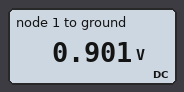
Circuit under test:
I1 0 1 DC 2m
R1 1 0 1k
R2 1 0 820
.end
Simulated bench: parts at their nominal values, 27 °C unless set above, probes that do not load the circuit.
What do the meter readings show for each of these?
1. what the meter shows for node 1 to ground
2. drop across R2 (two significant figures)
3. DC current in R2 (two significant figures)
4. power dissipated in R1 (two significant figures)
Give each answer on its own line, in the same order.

0.901 V
900 mV
1.1 mA
810 µW
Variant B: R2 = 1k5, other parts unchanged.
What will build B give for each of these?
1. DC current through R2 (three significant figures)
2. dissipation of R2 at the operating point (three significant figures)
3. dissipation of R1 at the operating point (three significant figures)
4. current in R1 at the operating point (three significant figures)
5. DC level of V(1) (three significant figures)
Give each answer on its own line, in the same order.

800 µA
960 µW
1.44 mW
1.20 mA
1.20 V
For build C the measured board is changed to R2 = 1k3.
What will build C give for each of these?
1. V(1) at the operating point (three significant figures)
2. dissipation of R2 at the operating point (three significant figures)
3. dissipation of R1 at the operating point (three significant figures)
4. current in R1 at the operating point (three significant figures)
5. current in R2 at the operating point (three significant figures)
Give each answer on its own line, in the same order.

1.13 V
983 µW
1.28 mW
1.13 mA
870 µA
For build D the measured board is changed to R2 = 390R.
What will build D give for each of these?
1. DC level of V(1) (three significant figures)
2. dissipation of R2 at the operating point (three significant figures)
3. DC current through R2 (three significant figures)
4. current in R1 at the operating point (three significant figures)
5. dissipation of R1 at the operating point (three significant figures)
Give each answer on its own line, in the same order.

561 mV
807 µW
1.44 mA
561 µA
315 µW
